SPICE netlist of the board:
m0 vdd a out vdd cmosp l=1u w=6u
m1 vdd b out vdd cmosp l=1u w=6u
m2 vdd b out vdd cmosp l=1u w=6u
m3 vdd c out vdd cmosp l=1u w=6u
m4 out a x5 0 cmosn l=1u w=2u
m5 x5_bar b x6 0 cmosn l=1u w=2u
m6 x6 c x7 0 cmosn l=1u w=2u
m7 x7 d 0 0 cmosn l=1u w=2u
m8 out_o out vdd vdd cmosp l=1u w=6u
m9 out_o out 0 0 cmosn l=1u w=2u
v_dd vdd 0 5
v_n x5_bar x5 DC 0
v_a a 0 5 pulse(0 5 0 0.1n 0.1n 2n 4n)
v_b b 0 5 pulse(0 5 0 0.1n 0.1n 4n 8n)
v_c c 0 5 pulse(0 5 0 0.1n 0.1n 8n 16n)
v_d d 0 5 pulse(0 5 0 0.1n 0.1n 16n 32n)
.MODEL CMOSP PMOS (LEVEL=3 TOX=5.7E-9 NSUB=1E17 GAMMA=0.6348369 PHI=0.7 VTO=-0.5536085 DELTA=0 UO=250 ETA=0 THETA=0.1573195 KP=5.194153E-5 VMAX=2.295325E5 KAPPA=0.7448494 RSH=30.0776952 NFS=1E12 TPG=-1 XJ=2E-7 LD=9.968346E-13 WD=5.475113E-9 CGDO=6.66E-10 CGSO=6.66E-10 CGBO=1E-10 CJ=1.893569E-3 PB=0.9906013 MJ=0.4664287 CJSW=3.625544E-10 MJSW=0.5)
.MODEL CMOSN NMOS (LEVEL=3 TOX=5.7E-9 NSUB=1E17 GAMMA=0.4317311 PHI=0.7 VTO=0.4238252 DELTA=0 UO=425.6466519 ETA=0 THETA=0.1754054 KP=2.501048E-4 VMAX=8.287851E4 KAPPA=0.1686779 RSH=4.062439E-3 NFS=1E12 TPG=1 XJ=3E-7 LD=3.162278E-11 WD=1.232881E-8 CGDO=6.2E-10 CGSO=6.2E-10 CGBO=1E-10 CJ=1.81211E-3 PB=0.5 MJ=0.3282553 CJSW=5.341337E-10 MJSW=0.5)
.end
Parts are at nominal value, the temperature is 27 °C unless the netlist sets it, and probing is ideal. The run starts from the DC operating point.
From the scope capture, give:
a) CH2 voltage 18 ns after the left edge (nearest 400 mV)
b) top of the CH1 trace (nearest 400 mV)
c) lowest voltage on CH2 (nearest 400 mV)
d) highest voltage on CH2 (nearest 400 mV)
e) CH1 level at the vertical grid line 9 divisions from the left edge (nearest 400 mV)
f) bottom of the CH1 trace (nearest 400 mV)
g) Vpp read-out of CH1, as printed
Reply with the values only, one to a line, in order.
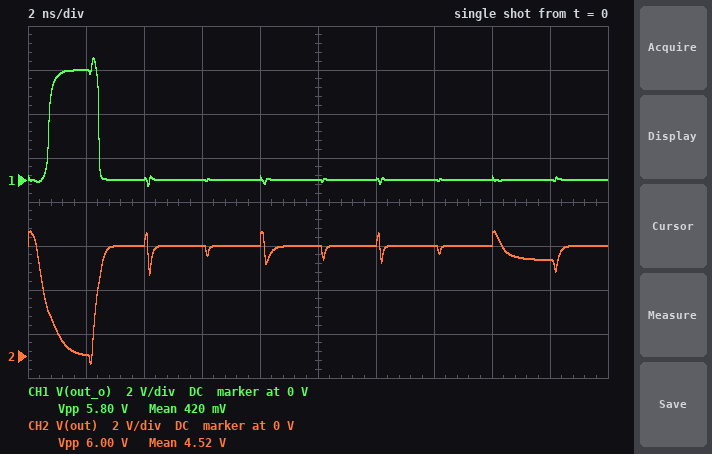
4.4 V
5.6 V
-400 mV
5.6 V
0 V
-400 mV
5.80 V
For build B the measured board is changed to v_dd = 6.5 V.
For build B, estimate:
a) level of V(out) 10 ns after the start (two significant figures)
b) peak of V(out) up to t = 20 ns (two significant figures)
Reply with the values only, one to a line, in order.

6.5 V
7.2 V
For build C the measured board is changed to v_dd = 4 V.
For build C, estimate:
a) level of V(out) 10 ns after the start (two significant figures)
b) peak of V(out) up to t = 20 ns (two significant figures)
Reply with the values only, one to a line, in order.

4.0 V
4.7 V
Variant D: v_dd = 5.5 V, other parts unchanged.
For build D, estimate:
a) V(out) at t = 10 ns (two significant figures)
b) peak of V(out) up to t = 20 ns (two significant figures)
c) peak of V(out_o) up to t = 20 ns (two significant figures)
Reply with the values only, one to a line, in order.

5.5 V
6.2 V
6.1 V
